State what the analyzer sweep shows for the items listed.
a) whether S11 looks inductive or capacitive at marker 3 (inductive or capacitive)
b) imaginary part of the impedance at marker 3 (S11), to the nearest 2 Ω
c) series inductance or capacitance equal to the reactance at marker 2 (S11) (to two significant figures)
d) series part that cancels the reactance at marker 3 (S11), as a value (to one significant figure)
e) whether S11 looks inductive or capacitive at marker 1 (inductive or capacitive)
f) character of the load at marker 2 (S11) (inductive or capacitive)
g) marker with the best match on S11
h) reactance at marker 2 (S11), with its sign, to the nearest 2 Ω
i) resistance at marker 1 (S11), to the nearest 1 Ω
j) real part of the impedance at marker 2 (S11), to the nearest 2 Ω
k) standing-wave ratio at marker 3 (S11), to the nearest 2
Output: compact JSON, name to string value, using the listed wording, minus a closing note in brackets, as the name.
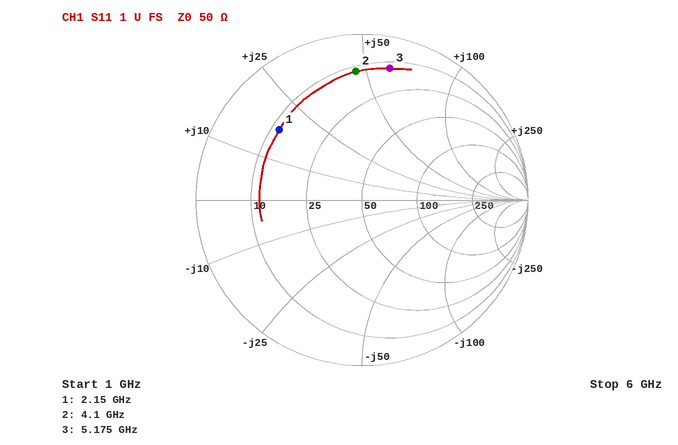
{"whether S11 looks inductive or capacitive at marker 3": "inductive", "imaginary part of the impedance at marker 3 (S11), to the nearest 2 Ω": "+60 Ω", "series inductance or capacitance equal to the reactance at marker 2 (S11)": "1.8 nH", "series part that cancels the reactance at marker 3 (S11), as a value": "500 fF", "whether S11 looks inductive or capacitive at marker 1": "inductive", "character of the load at marker 2 (S11)": "inductive", "marker with the best match on S11": "marker 1", "reactance at marker 2 (S11), with its sign, to the nearest 2 Ω": "+46 Ω", "resistance at marker 1 (S11), to the nearest 1 Ω": "12 Ω", "real part of the impedance at marker 2 (S11), to the nearest 2 Ω": "12 Ω", "standing-wave ratio at marker 3 (S11), to the nearest 2": "10"}
